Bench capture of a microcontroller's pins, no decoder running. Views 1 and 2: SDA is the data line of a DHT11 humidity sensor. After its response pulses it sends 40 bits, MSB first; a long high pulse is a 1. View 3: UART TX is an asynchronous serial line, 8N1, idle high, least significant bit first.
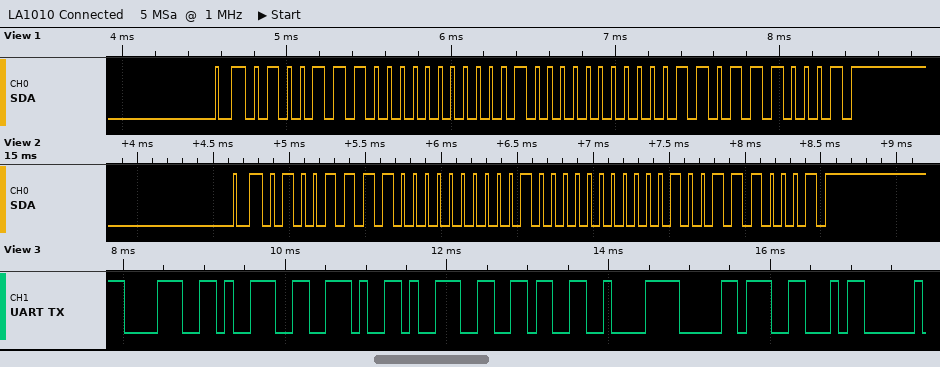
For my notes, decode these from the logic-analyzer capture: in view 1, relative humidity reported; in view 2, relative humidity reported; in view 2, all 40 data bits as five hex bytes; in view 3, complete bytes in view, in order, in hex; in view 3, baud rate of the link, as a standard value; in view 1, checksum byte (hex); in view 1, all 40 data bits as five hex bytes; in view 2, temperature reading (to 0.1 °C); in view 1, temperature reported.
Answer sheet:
78 %
79 %
4F 00 20 02 71
38 39 2E 39 36 C2 B0 46
9600 baud
0x71
4E 00 20 03 71
32.2 °C
32.3 °C
